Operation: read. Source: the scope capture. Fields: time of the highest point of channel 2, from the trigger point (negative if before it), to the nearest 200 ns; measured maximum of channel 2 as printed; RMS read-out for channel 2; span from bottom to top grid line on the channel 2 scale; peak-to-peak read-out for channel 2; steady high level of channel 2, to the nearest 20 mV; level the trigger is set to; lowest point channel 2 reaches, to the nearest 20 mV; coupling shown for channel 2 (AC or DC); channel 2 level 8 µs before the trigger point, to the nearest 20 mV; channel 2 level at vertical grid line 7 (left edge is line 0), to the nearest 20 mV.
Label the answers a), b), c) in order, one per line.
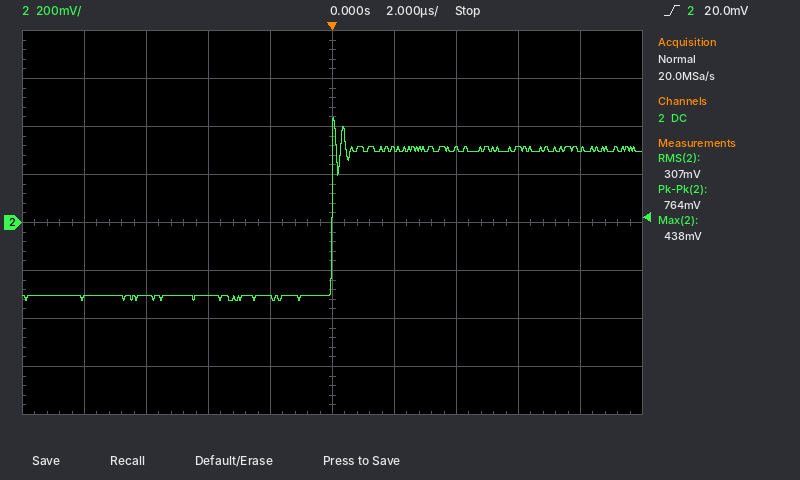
a) 0.0 µs
b) 438 mV
c) 307 mV
d) 1.6 V
e) 764 mV
f) 300 mV
g) 20.0 mV
h) -320 mV
i) DC
j) -320 mV
k) 300 mV
